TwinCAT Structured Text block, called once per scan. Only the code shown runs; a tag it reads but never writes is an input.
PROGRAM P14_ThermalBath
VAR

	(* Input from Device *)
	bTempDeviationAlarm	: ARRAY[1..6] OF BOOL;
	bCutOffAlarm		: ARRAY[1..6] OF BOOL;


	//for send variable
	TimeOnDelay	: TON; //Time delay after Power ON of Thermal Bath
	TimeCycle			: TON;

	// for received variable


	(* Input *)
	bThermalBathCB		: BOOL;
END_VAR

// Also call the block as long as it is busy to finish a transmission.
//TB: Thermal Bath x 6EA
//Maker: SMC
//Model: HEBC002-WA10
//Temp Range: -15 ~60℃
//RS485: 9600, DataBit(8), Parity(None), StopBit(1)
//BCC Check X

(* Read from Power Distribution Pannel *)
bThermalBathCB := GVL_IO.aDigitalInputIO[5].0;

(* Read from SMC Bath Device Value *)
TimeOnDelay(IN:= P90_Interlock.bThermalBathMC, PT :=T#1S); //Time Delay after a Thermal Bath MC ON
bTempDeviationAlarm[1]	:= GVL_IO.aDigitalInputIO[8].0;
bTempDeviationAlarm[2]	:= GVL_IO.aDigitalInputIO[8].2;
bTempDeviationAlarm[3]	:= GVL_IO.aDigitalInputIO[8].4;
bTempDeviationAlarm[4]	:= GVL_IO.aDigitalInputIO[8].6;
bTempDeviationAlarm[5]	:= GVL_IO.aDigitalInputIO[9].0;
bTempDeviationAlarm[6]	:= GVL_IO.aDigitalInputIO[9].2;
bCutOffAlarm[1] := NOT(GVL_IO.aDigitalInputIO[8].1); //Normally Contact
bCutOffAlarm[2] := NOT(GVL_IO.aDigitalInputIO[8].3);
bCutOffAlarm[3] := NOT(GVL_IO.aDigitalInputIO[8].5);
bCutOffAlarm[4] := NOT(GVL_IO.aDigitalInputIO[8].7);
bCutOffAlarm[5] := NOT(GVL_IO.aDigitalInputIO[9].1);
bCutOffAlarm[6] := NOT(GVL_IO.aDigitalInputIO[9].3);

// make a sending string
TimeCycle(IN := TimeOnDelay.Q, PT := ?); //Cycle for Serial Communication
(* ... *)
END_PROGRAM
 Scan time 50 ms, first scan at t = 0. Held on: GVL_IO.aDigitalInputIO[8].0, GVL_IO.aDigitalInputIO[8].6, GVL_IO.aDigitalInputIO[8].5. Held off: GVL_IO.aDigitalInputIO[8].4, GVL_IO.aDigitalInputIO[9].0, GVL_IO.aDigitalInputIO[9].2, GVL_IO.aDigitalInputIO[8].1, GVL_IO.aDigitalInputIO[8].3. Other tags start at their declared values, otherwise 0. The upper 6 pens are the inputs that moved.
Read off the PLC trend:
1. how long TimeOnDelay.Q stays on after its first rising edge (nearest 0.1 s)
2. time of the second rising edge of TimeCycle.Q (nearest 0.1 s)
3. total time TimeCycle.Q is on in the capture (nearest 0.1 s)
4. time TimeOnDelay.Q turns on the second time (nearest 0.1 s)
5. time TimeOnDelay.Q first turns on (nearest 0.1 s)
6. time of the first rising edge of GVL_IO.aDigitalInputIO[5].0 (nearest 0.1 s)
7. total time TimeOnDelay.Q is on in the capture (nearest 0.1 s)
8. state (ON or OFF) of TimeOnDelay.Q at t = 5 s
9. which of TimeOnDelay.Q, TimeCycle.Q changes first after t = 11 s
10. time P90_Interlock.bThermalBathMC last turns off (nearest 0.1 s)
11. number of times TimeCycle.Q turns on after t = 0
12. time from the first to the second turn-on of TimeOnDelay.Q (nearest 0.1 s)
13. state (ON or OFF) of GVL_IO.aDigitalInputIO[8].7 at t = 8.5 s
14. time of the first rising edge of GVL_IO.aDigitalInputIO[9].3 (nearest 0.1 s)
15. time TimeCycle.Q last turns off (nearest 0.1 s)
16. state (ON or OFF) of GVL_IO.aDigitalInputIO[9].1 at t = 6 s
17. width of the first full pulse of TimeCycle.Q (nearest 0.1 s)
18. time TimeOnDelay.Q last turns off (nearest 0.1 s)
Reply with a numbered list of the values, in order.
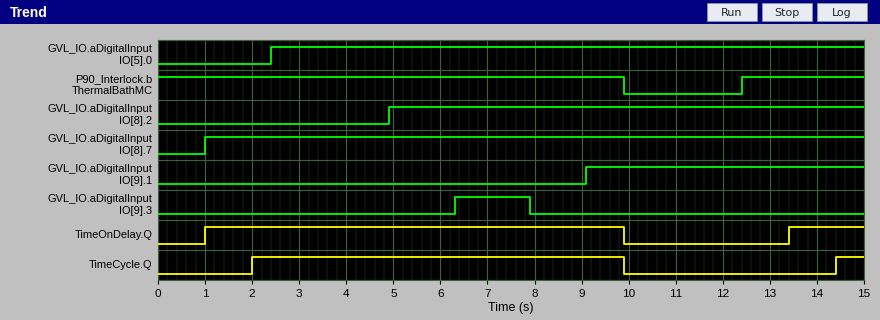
1. 8.9 s
2. 14.4 s
3. 8.5 s
4. 13.4 s
5. 1.0 s
6. 2.4 s
7. 10.5 s
8. ON
9. TimeOnDelay.Q
10. 9.9 s
11. 2
12. 12.4 s
13. ON
14. 6.3 s
15. 9.9 s
16. OFF
17. 7.9 s
18. 9.9 s
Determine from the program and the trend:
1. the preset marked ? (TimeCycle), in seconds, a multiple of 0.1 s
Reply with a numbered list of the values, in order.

1. 1.0 s
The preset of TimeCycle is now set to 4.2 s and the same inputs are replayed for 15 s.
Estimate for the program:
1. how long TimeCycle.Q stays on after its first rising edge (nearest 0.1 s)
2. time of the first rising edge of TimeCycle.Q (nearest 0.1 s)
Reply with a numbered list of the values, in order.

1. 4.7 s
2. 5.2 s
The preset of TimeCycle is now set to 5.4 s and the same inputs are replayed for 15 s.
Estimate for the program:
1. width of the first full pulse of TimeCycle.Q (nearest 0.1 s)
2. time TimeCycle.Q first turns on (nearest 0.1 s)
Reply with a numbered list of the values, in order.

1. 3.5 s
2. 6.4 s
